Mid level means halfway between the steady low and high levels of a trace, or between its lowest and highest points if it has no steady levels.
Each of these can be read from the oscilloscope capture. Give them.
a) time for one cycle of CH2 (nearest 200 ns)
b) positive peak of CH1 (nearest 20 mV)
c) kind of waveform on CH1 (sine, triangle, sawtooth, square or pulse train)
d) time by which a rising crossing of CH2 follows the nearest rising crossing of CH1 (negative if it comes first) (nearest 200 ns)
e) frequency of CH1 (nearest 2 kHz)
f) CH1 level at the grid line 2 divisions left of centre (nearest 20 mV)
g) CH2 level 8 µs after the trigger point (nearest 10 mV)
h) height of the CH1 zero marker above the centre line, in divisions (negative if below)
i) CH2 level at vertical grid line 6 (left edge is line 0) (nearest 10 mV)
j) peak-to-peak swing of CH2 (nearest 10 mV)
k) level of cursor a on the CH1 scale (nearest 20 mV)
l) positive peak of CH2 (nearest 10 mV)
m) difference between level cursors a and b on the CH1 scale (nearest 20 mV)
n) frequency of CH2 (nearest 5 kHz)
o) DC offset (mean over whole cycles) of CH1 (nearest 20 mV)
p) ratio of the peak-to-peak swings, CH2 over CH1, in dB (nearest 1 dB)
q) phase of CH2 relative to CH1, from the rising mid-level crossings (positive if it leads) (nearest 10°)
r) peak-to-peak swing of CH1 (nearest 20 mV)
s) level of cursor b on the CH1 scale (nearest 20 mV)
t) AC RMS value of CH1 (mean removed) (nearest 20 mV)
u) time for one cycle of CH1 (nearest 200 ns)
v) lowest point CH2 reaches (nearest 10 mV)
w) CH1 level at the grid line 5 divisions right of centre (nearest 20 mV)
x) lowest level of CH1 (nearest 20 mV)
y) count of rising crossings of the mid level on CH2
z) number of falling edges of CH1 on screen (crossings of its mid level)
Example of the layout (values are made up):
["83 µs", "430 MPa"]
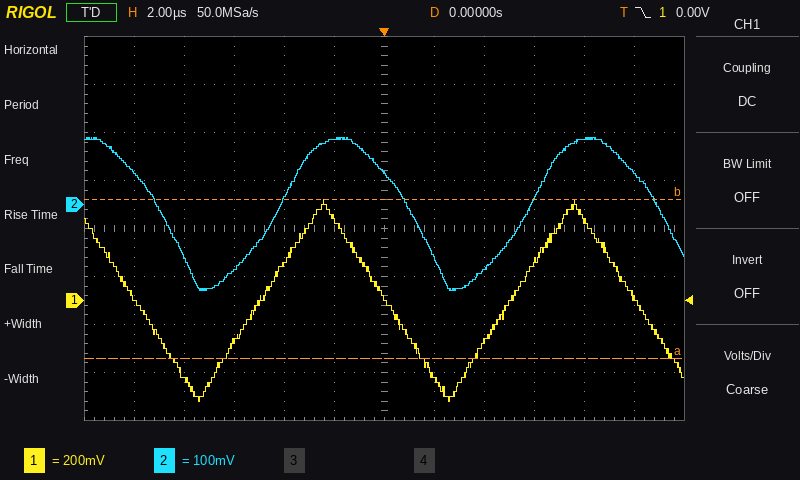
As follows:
["10.0 µs", "420 mV", "triangle", "+600 ns", "100 kHz", "160 mV", "140 mV", "-1.5 div", "60 mV", "320 mV", "-240 mV", "140 mV", "660 mV", "100 kHz", "0 mV", "-8 dB", "-20°", "840 mV", "420 mV", "240 mV", "10.0 µs", "-180 mV", "20 mV", "-420 mV", "2", "3"]
